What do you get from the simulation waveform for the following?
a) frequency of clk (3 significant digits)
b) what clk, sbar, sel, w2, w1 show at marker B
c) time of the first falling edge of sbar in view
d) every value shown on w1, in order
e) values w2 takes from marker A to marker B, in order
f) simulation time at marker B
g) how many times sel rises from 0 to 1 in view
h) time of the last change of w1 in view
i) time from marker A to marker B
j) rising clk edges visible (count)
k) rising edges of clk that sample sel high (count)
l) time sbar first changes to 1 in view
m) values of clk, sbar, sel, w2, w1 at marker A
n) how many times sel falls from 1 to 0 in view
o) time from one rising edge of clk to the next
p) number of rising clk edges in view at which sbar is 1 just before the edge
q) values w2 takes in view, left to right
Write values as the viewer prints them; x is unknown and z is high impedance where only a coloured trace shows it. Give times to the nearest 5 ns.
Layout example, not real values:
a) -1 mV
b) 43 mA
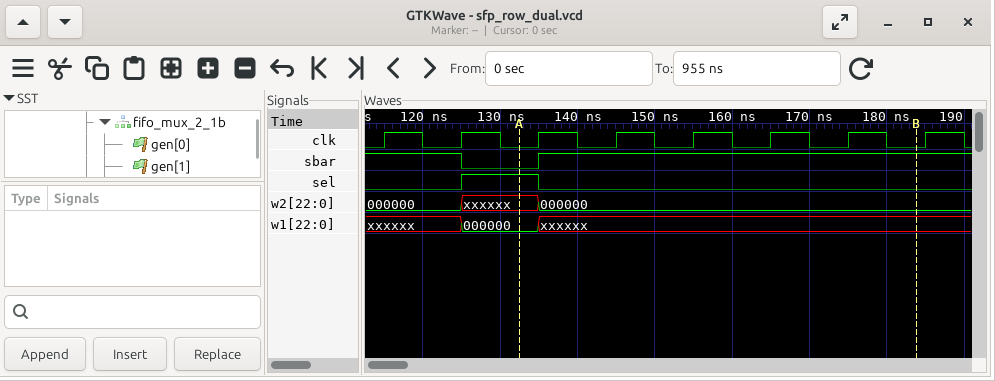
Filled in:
a) 100 MHz
b) clk=0, sbar=1, sel=0, w2=000000, w1=xxxxxx
c) 125 ns
d) xxxxxx, 000000, xxxxxx
e) xxxxxx, 000000
f) 185 ns
g) 1
h) 135 ns
i) 50 ns
j) 8
k) 1
l) 135 ns
m) clk=0, sbar=0, sel=1, w2=xxxxxx, w1=000000
n) 1
o) 10 ns
p) 7
q) 000000, xxxxxx, 000000
